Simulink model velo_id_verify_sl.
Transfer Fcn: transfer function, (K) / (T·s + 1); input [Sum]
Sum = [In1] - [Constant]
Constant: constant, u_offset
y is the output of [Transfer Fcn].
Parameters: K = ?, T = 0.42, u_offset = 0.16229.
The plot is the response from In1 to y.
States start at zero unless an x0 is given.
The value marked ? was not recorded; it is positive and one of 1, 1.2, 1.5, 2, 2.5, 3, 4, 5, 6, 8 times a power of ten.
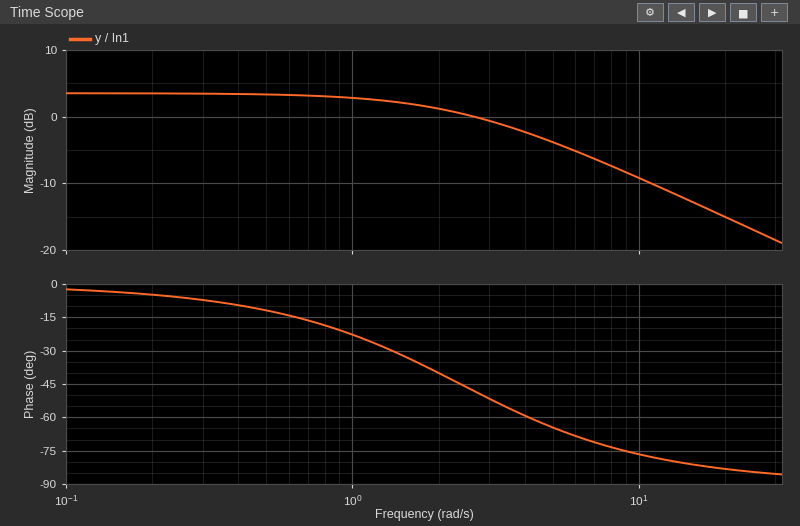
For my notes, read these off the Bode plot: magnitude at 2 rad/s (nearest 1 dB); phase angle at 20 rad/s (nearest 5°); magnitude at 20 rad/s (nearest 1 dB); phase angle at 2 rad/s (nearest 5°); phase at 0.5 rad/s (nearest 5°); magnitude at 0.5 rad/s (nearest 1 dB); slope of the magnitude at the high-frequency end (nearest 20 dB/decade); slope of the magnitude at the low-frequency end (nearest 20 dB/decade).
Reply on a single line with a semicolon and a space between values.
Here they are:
1 dB; -85°; -15 dB; -40°; -10°; 3 dB; -20 dB/decade; 0 dB/decade
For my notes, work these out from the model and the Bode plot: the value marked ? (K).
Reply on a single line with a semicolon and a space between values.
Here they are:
1.5
